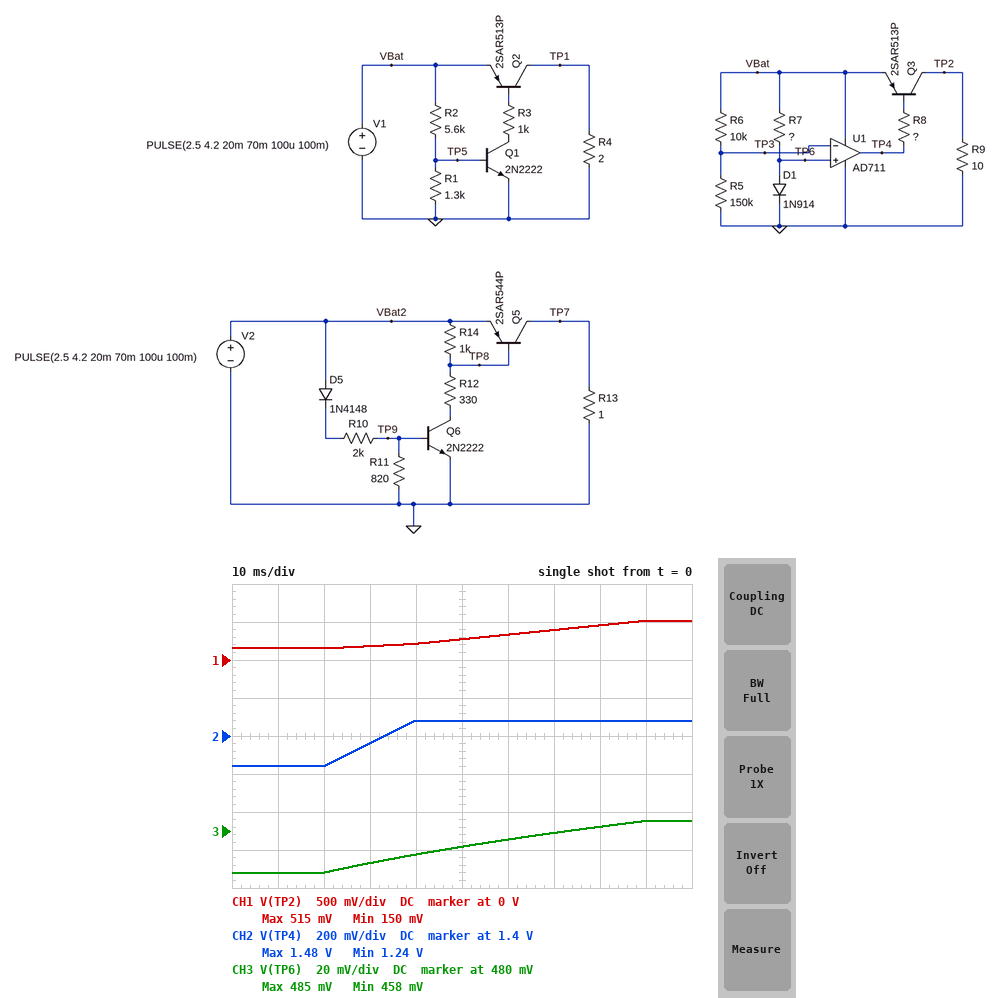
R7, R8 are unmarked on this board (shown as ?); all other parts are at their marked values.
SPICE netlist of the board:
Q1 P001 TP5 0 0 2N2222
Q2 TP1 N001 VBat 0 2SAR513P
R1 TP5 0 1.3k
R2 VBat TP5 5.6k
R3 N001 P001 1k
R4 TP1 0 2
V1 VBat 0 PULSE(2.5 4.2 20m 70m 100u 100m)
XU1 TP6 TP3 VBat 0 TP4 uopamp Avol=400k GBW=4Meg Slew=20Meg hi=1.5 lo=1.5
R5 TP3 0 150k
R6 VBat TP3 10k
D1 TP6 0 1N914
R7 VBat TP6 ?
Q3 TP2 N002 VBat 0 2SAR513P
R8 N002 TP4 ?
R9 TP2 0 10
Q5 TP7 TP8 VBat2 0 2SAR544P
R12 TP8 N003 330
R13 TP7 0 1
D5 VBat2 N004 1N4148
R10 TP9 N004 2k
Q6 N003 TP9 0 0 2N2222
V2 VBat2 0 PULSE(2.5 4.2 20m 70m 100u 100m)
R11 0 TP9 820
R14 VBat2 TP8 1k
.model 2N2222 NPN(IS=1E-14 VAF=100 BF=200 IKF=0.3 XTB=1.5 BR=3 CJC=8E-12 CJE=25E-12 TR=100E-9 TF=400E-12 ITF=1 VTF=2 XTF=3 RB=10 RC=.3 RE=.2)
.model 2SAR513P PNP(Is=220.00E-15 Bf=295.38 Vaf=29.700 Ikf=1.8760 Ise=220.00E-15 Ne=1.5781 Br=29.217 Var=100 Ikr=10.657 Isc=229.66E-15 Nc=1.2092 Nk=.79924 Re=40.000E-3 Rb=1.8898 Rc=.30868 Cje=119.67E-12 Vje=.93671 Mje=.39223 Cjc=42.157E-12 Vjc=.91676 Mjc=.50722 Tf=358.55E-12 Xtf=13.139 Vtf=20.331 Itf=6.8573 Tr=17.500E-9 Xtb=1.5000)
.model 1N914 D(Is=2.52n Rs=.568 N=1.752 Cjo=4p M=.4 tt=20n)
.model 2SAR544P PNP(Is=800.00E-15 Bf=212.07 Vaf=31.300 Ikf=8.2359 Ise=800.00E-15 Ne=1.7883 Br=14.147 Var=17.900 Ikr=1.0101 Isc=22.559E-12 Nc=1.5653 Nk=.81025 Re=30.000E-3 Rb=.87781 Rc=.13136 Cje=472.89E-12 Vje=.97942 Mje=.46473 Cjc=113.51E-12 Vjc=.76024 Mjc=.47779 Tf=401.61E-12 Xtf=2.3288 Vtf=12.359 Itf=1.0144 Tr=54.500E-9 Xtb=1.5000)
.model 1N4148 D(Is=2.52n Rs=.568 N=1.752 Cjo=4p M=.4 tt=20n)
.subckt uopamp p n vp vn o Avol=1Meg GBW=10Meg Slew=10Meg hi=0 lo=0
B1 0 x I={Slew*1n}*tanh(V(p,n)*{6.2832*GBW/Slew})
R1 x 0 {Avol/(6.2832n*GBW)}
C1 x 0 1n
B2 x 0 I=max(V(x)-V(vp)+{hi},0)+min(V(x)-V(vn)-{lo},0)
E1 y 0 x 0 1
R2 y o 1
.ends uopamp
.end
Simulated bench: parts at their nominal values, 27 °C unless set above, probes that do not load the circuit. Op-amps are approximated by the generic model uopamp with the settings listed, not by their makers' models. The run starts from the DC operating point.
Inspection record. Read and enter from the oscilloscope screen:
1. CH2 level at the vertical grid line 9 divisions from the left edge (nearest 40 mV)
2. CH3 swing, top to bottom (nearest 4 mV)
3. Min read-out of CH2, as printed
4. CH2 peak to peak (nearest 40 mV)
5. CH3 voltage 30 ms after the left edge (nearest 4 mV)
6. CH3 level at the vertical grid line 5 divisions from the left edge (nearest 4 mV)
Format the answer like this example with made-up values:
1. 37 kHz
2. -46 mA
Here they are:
1. 1.48 V
2. 28 mV
3. 1.24 V
4. 240 mV
5. 464 mV
6. 472 mV
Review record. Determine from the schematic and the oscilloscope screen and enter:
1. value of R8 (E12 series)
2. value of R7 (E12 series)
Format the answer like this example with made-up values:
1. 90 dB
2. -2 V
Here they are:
1. 12 kΩ
2. 33 kΩ
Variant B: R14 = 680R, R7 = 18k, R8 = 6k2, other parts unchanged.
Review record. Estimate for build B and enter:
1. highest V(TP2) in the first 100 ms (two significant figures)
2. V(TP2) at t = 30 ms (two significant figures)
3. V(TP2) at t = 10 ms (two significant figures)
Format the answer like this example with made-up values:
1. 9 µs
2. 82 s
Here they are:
1. 950 mV
2. 340 mV
3. 280 mV
